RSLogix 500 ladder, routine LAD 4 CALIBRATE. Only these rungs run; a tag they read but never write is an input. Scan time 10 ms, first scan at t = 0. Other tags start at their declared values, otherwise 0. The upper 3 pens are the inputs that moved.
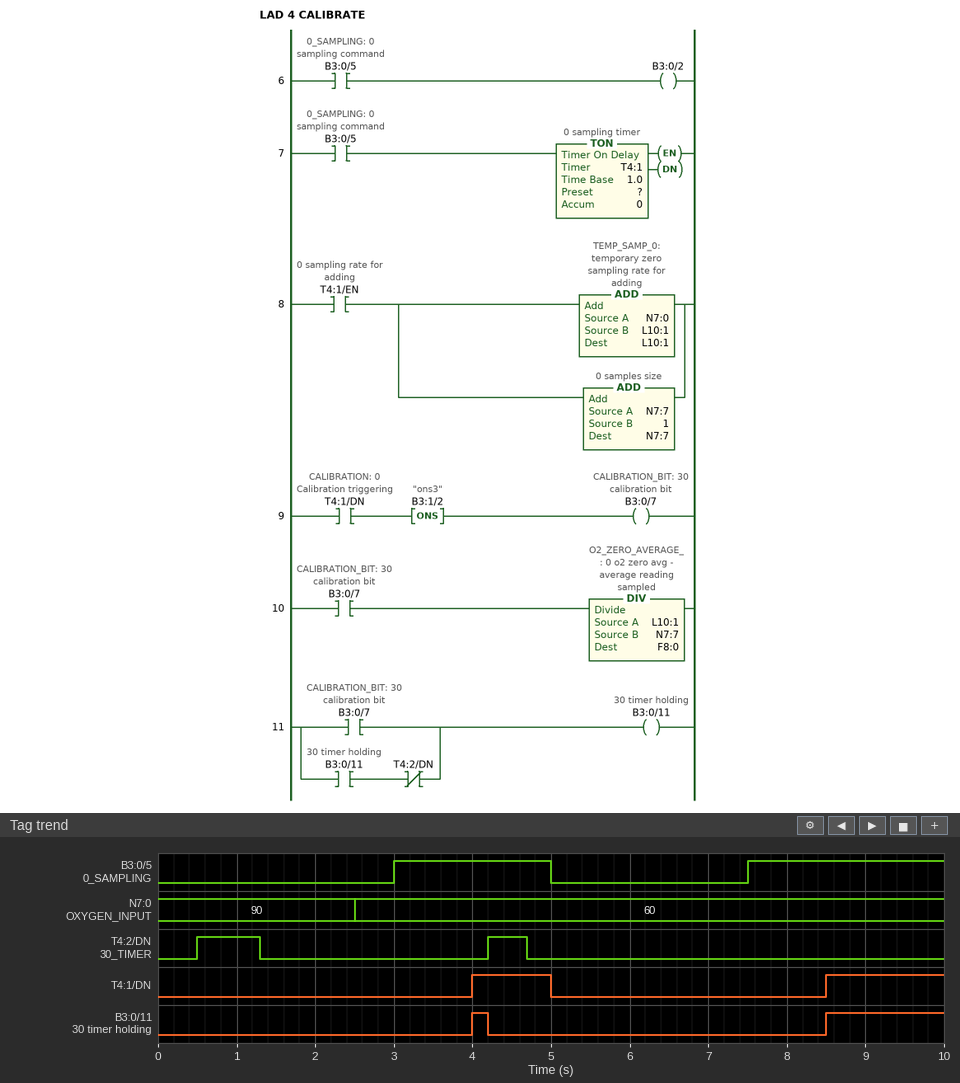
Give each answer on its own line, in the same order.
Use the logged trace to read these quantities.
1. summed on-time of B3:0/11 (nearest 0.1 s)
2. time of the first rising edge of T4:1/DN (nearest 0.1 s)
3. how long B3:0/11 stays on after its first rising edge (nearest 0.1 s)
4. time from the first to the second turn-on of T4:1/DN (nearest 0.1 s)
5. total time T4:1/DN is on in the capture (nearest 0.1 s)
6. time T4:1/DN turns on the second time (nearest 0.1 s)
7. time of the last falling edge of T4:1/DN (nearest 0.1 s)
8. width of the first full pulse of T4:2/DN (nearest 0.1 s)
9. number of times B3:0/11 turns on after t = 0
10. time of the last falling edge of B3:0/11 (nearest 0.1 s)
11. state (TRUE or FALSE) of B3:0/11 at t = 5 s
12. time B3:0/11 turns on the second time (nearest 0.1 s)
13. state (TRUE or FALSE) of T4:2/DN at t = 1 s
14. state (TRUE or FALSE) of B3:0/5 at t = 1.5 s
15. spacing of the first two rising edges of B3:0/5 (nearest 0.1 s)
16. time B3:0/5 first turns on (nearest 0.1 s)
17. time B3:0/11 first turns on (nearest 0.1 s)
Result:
1.7 s
4.0 s
0.2 s
4.5 s
2.5 s
8.5 s
5.0 s
0.8 s
2
4.2 s
FALSE
8.5 s
TRUE
FALSE
4.5 s
3.0 s
4.0 s
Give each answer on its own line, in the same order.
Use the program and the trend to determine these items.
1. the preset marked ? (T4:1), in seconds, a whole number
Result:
1 s
